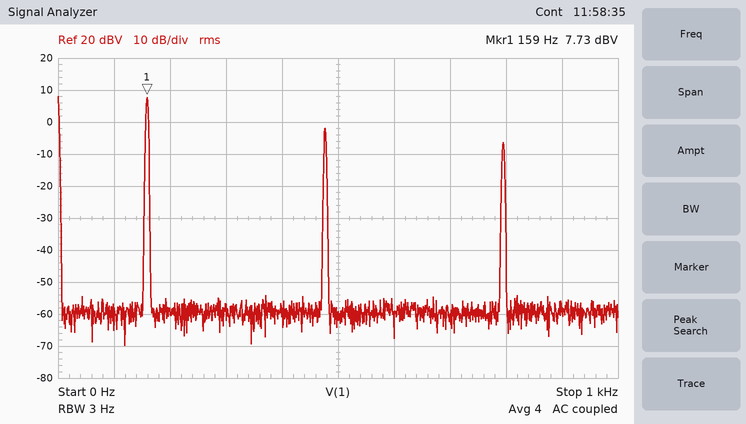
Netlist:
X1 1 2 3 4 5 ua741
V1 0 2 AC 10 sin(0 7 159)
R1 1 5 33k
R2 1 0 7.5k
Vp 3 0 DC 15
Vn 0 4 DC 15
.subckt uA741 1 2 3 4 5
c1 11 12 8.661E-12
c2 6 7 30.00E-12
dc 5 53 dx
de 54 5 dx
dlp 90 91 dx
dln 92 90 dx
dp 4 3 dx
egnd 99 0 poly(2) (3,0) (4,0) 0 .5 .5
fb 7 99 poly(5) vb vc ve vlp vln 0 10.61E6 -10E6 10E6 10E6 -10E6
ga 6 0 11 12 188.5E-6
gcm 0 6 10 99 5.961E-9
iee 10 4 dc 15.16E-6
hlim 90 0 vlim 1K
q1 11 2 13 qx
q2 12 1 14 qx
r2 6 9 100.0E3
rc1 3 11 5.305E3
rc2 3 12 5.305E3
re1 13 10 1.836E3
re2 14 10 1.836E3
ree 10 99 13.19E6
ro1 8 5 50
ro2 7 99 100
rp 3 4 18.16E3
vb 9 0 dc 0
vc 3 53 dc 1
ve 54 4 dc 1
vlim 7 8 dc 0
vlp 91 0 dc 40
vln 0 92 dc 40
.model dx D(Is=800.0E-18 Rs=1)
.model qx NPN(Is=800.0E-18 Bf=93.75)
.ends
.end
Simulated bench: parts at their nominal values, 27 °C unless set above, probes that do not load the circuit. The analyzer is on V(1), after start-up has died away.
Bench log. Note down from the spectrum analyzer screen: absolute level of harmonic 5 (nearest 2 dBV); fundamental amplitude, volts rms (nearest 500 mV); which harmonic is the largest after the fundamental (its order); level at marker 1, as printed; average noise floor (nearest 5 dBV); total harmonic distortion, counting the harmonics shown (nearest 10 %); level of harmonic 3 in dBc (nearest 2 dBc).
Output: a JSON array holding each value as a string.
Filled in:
["-6 dBV", "2.5 V", "3", "7.73 dBV", "-60 dBV", "40 %", "-10 dBc"]
